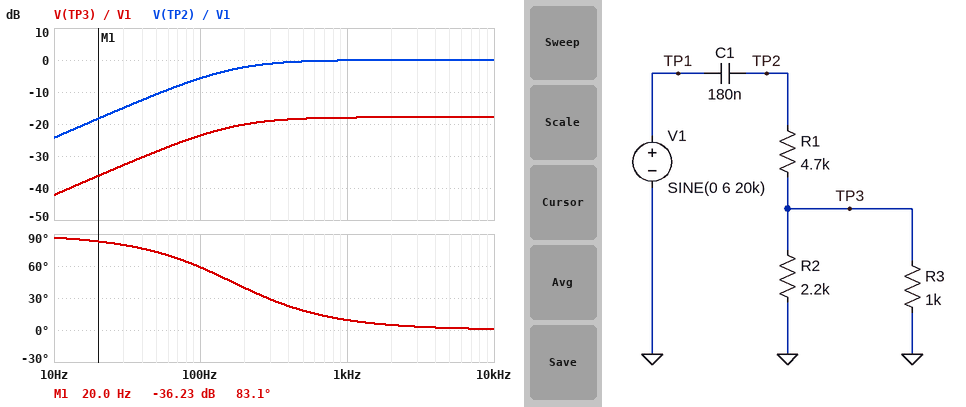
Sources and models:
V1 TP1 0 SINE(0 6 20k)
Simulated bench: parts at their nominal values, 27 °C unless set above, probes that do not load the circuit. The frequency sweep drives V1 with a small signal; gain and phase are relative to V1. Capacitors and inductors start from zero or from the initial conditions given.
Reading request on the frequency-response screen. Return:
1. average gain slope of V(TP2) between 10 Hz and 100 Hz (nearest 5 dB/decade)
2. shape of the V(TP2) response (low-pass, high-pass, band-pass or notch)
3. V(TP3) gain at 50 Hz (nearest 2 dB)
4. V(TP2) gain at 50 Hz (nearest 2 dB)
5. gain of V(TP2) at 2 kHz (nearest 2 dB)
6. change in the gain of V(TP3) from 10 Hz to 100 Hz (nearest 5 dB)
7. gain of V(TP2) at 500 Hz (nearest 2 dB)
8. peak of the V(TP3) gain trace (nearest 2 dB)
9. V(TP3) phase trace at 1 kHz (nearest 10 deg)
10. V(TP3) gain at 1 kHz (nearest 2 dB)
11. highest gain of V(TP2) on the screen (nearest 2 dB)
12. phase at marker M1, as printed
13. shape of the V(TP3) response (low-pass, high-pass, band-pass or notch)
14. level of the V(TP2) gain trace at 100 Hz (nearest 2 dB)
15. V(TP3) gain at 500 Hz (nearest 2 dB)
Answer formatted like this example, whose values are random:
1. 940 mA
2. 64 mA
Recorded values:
1. 20 dB/decade
2. high-pass
3. -28 dB
4. -10 dB
5. 0 dB
6. 20 dB
7. 0 dB
8. -18 dB
9. 10 deg
10. -18 dB
11. 0 dB
12. 83.1 deg
13. high-pass
14. -6 dB
15. -18 dB
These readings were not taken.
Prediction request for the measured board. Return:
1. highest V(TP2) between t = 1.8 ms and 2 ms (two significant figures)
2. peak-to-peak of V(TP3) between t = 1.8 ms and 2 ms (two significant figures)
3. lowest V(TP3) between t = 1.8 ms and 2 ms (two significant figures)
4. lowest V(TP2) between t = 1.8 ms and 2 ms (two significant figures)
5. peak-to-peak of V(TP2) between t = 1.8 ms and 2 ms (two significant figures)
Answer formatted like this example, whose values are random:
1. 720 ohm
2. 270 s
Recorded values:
1. 6.0 V
2. 1.5 V
3. -770 mV
4. -6.0 V
5. 12 V
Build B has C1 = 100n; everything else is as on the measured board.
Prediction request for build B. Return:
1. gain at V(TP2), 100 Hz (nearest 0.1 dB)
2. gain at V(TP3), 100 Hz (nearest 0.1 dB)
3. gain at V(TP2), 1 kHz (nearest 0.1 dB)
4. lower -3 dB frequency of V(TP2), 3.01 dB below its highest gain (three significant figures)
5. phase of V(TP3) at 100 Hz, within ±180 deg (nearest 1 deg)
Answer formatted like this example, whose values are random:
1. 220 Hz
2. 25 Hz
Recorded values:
1. -9.9 dB
2. -27.8 dB
3. -0.4 dB
4. 295 Hz
5. 71 deg
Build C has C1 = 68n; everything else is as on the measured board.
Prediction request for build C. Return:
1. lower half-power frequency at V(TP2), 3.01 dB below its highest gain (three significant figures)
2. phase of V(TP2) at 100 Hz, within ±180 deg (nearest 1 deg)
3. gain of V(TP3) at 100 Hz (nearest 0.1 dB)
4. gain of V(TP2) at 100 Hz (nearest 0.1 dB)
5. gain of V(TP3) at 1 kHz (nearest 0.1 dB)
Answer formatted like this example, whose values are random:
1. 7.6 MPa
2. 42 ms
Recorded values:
1. 434 Hz
2. 77 deg
3. -30.9 dB
4. -13.0 dB
5. -18.6 dB
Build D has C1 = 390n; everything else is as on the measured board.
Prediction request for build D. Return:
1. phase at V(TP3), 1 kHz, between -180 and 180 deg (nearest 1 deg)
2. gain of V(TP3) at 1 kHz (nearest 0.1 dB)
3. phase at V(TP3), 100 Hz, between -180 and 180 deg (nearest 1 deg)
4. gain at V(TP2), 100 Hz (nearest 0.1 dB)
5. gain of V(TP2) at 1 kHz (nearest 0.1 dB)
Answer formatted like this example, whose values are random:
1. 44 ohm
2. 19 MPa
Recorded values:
1. 4 deg
2. -17.9 dB
3. 37 deg
4. -2.0 dB
5. 0 dB
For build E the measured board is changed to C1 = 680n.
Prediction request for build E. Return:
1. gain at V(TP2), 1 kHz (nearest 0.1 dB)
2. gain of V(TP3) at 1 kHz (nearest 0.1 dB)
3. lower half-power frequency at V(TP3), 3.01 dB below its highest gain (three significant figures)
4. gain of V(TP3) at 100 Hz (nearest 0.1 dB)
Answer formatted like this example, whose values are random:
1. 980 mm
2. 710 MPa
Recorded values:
1. 0 dB
2. -17.9 dB
3. 43.4 Hz
4. -18.6 dB
